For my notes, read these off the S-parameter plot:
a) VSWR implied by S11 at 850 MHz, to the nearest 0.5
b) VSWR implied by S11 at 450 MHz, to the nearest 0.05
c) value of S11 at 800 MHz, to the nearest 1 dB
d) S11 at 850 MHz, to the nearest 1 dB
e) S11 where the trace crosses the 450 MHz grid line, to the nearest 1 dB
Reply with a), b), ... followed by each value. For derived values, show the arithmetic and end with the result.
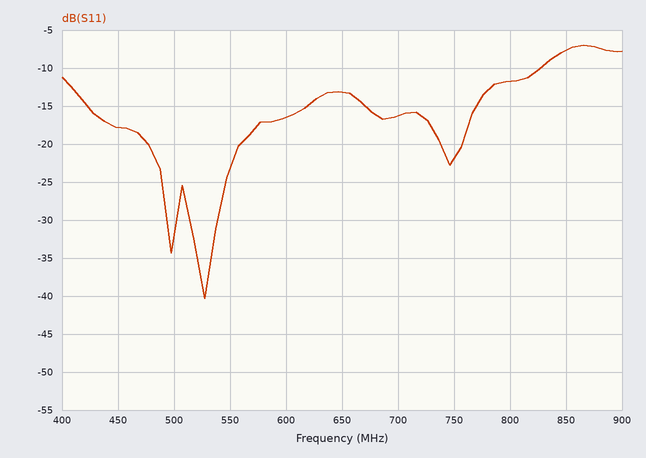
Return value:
a) |Γ| = 10^(-8/20) = 0.3981; VSWR = (1 + 0.3981)/(1 − 0.3981) ≈ 2.32, so 2.5 to the nearest 0.5
b) |Γ| = 10^(-18/20) = 0.1259; VSWR = (1 + 0.1259)/(1 − 0.1259) ≈ 1.29, so 1.30 to the nearest 0.05
c) -12 dB
d) -8 dB
e) -18 dB
